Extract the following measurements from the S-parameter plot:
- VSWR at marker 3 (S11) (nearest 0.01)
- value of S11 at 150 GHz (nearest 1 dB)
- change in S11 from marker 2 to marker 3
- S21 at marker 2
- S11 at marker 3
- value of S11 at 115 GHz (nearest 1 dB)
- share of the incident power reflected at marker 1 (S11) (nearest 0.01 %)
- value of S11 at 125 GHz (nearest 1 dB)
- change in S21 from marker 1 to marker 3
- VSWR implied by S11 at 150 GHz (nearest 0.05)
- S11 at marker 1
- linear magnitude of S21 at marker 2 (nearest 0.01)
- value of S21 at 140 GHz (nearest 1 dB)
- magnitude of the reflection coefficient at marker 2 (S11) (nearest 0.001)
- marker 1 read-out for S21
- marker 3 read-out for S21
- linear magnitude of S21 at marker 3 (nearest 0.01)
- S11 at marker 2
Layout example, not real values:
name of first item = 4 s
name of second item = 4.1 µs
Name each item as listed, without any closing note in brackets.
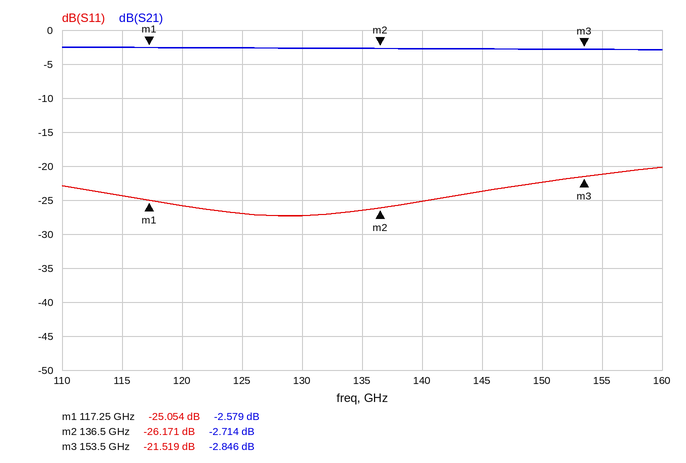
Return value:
VSWR at marker 3 (S11) = 1.18
value of S11 at 150 GHz = -22 dB
change in S11 from marker 2 to marker 3 = 4.652 dB
S21 at marker 2 = -2.714 dB
S11 at marker 3 = -21.519 dB
value of S11 at 115 GHz = -24 dB
share of the incident power reflected at marker 1 (S11) = 0.31 %
value of S11 at 125 GHz = -27 dB
change in S21 from marker 1 to marker 3 = -0.267 dB
VSWR implied by S11 at 150 GHz = 1.15
S11 at marker 1 = -25.054 dB
linear magnitude of S21 at marker 2 = 0.73
value of S21 at 140 GHz = -3 dB
magnitude of the reflection coefficient at marker 2 (S11) = 0.049
marker 1 read-out for S21 = -2.579 dB
marker 3 read-out for S21 = -2.846 dB
linear magnitude of S21 at marker 3 = 0.72
S11 at marker 2 = -26.171 dB
